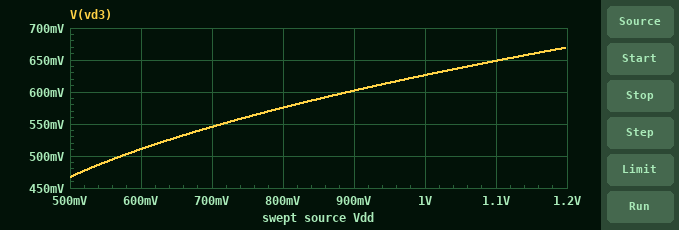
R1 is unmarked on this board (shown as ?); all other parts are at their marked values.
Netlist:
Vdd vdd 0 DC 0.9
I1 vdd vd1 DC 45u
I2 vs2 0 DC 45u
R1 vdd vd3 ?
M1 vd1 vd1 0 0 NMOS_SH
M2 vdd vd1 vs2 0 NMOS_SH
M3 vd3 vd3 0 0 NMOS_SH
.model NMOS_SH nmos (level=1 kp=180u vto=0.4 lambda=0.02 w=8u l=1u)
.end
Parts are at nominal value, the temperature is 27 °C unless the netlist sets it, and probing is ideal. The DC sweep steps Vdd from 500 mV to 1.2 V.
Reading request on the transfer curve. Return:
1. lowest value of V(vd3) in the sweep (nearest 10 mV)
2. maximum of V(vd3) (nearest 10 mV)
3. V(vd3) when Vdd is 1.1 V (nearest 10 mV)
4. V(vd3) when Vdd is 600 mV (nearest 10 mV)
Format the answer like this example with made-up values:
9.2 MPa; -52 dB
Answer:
470 mV; 670 mV; 650 mV; 510 mV
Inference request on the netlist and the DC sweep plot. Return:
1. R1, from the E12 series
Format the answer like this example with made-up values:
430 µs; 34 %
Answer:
10 kΩ
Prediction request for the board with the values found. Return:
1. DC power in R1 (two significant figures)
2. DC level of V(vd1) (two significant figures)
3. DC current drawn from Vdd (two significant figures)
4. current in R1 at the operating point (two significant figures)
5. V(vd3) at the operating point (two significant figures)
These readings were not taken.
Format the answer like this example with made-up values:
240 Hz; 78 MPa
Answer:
8.9 µW; 650 mV; 120 µA; 30 µA; 600 mV
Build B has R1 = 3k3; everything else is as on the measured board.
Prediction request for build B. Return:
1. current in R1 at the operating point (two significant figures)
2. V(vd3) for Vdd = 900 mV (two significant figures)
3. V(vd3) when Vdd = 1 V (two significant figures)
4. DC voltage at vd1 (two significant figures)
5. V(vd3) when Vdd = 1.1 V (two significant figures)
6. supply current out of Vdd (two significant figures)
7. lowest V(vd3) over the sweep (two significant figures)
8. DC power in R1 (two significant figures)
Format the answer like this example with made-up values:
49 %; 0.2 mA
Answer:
63 µA; 690 mV; 730 mV; 650 mV; 770 mV; 150 µA; 480 mV; 13 µW
